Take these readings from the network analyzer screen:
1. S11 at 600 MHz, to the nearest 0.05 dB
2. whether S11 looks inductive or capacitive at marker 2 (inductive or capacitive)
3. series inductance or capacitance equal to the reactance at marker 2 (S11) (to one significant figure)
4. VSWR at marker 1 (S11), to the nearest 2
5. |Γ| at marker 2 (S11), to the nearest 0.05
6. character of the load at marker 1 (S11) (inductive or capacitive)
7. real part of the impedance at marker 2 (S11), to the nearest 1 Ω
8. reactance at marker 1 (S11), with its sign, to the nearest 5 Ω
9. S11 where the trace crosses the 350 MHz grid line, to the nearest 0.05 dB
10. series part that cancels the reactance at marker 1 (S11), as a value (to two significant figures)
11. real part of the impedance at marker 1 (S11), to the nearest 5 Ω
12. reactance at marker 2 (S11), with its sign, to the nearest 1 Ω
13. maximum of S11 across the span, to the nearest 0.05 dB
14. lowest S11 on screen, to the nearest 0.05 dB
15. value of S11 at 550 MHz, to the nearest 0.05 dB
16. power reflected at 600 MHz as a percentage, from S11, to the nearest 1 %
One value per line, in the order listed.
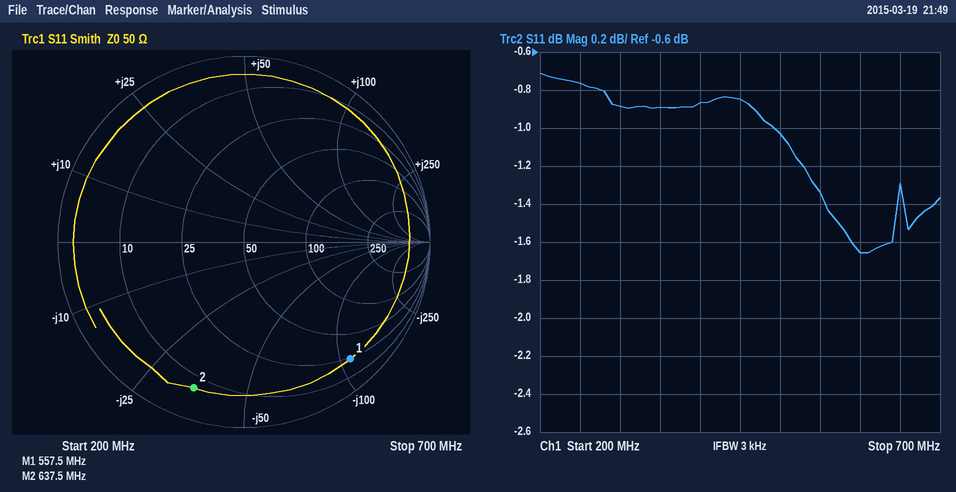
-1.65 dB
capacitive
7 pF
12
0.85
capacitive
7 Ω
-110 Ω
-0.90 dB
31 nH
25 Ω
-35 Ω
-0.70 dB
-1.65 dB
-1.35 dB
68 %
